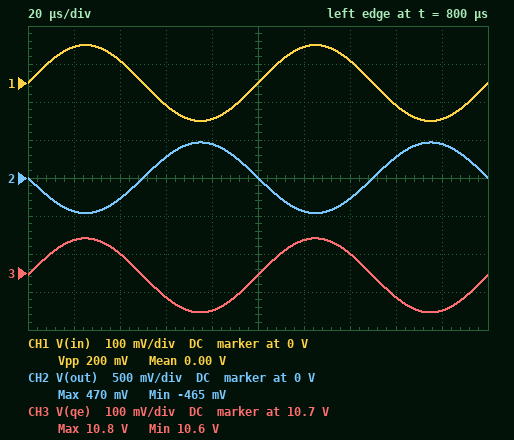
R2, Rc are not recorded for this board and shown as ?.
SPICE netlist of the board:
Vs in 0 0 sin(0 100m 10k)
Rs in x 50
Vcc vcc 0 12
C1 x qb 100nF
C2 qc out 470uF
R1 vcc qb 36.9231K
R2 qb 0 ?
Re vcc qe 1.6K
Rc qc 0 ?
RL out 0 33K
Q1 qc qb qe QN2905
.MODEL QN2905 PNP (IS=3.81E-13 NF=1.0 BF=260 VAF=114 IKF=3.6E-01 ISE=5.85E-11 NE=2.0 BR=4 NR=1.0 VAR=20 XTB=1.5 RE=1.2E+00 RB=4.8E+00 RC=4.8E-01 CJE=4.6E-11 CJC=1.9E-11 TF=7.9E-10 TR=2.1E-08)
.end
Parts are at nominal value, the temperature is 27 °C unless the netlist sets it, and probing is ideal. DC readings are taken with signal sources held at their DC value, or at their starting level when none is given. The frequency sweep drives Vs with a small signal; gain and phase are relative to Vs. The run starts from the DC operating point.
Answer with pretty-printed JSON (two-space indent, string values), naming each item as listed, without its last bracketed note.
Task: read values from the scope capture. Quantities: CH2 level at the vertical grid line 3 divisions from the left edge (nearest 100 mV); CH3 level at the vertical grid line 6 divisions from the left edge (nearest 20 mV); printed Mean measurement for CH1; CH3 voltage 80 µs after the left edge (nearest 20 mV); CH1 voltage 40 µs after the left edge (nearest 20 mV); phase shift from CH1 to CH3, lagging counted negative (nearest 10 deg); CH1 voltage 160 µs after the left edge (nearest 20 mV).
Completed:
{
  "CH2 level at the vertical grid line 3 divisions from the left edge": "300 mV",
  "CH3 level at the vertical grid line 6 divisions from the left edge": "10.78 V",
  "printed Mean measurement for CH1": "0.00 V",
  "CH3 voltage 80 µs after the left edge": "10.60 V",
  "CH1 voltage 40 µs after the left edge": "60 mV",
  "phase shift from CH1 to CH3, lagging counted negative": "0 deg",
  "CH1 voltage 160 µs after the left edge": "-60 mV"
}
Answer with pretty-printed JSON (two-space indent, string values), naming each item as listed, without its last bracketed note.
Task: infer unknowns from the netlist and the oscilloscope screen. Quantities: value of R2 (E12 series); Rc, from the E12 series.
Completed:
{
  "value of R2": "180 kΩ",
  "Rc, from the E12 series": "10 kΩ"
}
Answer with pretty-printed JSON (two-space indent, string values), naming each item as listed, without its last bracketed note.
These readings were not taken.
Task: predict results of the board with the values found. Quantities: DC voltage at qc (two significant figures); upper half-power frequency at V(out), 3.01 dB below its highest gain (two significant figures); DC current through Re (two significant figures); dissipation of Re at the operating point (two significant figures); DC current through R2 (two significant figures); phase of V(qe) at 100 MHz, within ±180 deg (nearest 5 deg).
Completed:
{
  "DC voltage at qc": "8.1 V",
  "upper half-power frequency at V(out), 3.01 dB below its highest gain": "1.7 MHz",
  "DC current through Re": "820 µA",
  "dissipation of Re at the operating point": "1.1 mW",
  "DC current through R2": "56 µA",
  "phase of V(qe) at 100 MHz, within ±180 deg": "0 deg"
}
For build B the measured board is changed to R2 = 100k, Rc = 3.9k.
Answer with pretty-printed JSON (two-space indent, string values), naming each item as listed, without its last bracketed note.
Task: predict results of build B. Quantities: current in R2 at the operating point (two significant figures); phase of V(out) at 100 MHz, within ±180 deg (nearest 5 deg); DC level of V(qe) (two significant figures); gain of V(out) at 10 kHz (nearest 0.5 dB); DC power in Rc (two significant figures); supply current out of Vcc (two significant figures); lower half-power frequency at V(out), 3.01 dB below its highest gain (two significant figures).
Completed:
{
  "current in R2 at the operating point": "90 µA",
  "phase of V(out) at 100 MHz, within ±180 deg": "5 deg",
  "DC level of V(qe)": "9.6 V",
  "gain of V(out) at 10 kHz": "6.5 dB",
  "DC power in Rc": "8.7 mW",
  "supply current out of Vcc": "1.6 mA",
  "lower half-power frequency at V(out), 3.01 dB below its highest gain": "64 Hz"
}
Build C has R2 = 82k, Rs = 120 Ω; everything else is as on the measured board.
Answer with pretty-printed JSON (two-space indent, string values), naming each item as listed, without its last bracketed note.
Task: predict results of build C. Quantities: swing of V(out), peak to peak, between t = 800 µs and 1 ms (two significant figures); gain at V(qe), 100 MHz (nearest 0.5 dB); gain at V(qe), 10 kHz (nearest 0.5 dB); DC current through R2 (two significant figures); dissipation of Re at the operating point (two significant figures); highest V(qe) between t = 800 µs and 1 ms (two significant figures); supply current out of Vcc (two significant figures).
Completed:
{
  "swing of V(out), peak to peak, between t = 800 µs and 1 ms": "89 mV",
  "gain at V(qe), 100 MHz": "-1.0 dB",
  "gain at V(qe), 10 kHz": "-1.5 dB",
  "DC current through R2": "120 µA",
  "dissipation of Re at the operating point": "1.9 mW",
  "highest V(qe) between t = 800 µs and 1 ms": "10 V",
  "supply current out of Vcc": "1.1 mA"
}
